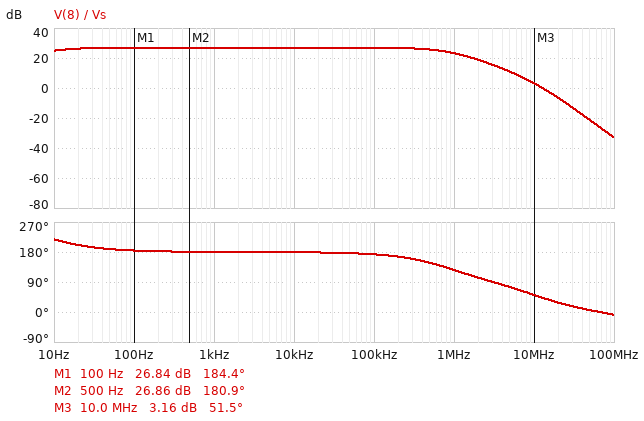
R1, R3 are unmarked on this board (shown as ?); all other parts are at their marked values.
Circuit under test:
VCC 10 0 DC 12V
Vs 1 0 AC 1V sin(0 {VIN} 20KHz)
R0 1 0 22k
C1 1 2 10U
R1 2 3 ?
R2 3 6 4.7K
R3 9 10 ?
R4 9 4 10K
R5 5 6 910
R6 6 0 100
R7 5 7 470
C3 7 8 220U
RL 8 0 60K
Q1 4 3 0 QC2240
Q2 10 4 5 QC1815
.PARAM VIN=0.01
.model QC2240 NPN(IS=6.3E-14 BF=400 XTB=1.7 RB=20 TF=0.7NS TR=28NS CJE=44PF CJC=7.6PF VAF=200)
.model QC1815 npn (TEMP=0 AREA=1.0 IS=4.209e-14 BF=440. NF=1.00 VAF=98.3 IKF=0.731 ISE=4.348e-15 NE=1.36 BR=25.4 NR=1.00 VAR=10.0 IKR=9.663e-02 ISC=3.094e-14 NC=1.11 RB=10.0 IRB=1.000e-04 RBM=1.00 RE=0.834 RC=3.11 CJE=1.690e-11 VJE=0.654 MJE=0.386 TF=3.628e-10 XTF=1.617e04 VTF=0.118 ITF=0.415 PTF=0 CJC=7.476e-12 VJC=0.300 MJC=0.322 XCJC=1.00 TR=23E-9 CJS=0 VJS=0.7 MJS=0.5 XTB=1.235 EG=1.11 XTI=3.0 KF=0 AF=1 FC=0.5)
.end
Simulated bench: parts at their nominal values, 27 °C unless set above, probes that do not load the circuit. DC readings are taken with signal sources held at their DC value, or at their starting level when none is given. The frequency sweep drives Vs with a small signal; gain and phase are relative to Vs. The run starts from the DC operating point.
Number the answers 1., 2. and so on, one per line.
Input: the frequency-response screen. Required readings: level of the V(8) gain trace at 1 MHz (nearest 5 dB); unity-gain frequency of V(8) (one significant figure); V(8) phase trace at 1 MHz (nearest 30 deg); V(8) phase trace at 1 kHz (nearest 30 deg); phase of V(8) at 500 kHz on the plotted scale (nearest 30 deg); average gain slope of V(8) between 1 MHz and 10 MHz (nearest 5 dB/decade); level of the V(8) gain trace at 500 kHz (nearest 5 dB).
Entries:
1. 25 dB
2. 10 MHz
3. 120 deg
4. 180 deg
5. 150 deg
6. -20 dB/decade
7. 25 dB
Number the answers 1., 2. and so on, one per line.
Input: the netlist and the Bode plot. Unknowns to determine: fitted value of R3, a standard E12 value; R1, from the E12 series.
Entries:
1. 15 kΩ
2. 1.8 kΩ
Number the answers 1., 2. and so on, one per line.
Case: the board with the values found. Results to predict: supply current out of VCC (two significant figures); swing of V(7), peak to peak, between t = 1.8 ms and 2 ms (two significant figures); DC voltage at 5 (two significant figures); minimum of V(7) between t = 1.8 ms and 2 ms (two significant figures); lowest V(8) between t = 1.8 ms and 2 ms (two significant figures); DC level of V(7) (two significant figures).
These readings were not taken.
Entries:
1. 5.9 mA
2. 440 mV
3. 5.7 V
4. 5.5 V
5. -220 mV
6. 5.7 V
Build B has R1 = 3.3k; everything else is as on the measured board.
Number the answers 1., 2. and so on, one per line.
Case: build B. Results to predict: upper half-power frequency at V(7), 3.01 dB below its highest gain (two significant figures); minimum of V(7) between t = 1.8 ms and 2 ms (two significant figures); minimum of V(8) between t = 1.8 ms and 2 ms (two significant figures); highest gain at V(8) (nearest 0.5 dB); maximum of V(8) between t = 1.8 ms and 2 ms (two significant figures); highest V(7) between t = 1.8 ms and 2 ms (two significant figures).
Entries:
1. 870 kHz
2. 5.6 V
3. -130 mV
4. 22.0 dB
5. 130 mV
6. 5.9 V
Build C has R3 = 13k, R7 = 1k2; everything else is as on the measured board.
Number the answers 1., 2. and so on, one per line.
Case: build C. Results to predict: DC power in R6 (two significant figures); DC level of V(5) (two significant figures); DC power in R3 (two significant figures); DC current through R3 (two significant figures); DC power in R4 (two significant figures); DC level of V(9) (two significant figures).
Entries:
1. 3.3 mW
2. 5.8 V
3. 750 µW
4. 240 µA
5. 580 µW
6. 8.9 V
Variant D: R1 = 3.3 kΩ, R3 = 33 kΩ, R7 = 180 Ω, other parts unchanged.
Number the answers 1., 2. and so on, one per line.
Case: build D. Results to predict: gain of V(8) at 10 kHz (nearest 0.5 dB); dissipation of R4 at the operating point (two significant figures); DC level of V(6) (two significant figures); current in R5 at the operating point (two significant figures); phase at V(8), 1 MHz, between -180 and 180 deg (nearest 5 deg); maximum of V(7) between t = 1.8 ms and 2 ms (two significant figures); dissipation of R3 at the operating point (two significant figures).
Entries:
1. 22.0 dB
2. 180 µW
3. 550 mV
4. 5.5 mA
5. 120 deg
6. 5.7 V
7. 580 µW
